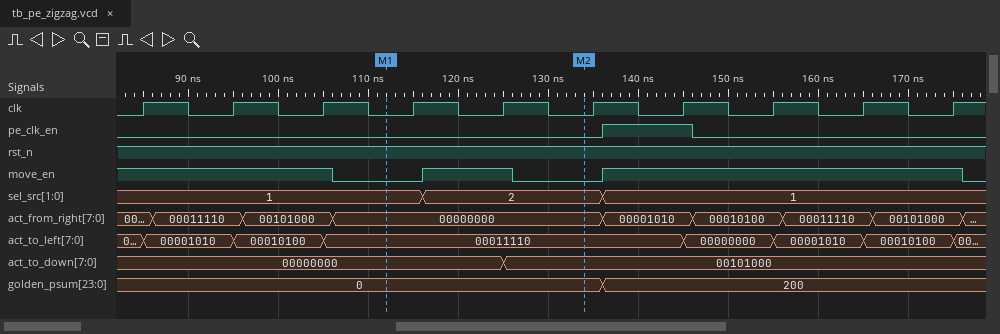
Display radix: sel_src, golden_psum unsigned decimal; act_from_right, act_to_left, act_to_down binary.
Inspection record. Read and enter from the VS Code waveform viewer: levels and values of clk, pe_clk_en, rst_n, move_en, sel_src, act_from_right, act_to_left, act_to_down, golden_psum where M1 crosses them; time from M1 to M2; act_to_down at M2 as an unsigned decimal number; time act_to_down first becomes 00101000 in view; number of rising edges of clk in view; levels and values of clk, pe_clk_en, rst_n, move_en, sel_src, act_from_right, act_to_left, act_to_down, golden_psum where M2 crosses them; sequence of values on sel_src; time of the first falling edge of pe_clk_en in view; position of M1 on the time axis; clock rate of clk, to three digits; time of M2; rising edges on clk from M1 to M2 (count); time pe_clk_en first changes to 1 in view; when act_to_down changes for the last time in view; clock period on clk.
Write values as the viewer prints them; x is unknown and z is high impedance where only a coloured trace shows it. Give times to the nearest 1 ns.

clk=0, pe_clk_en=0, rst_n=1, move_en=0, sel_src=1, act_from_right=00000000, act_to_left=00011110, act_to_down=00000000, golden_psum=0
22 ns
40
125 ns
10
clk=0, pe_clk_en=0, rst_n=1, move_en=0, sel_src=2, act_from_right=00000000, act_to_left=00011110, act_to_down=00101000, golden_psum=0
1, 2, 1
146 ns
112 ns
100 MHz
134 ns
2
136 ns
125 ns
10 ns
